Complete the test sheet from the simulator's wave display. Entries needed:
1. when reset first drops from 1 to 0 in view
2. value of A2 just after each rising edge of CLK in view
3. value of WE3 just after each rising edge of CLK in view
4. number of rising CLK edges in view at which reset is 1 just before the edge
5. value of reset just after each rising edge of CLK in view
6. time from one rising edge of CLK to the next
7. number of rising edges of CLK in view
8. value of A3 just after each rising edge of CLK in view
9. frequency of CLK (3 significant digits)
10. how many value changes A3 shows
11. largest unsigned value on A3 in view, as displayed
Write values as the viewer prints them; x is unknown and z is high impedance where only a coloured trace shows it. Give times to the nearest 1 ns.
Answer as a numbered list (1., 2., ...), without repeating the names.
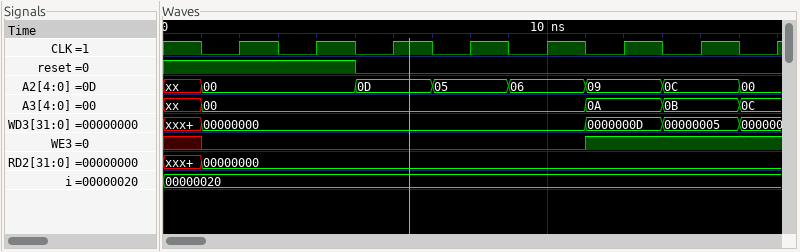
1. 5 ns
2. 00, 00, 0D, 05, 06, 09, 0C, 00
3. 0 0 0 0 0 1 1 1
4. 2
5. 1 1 0 0 0 0 0 0
6. 2 ns
7. 8
8. 00, 00, 00, 00, 00, 0A, 0B, 0C
9. 500 MHz
10. 4
11. 0C
